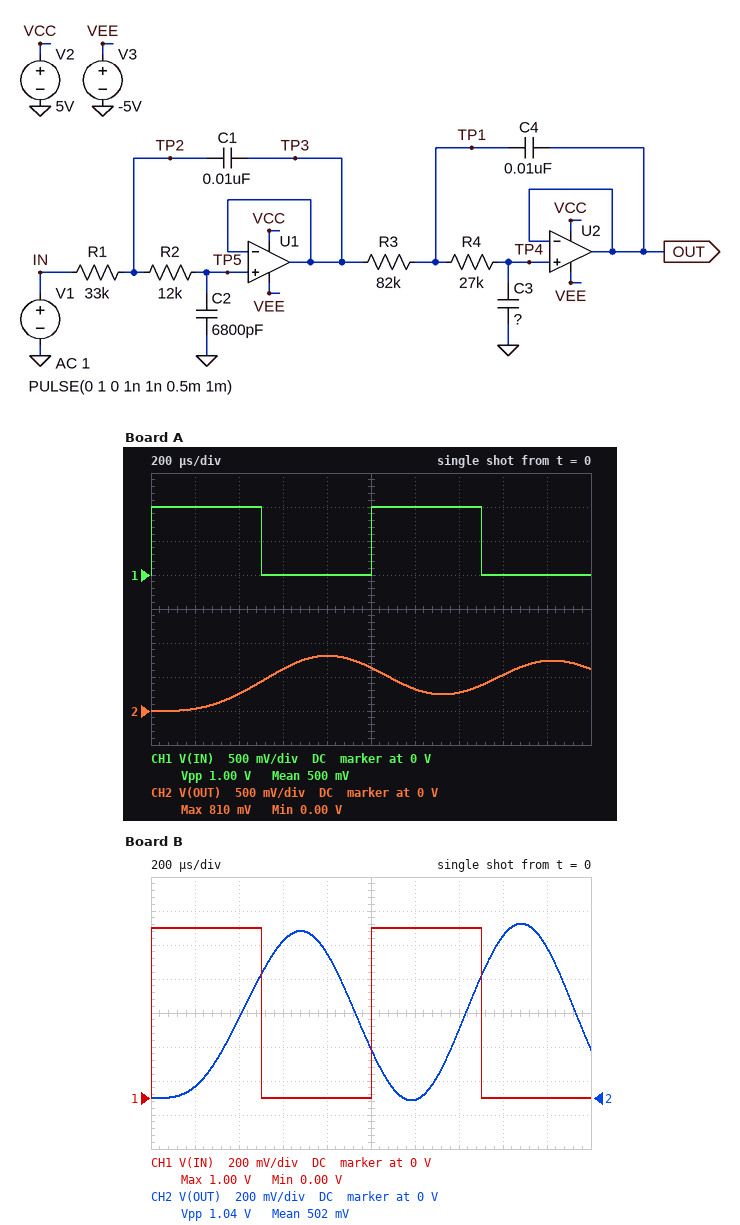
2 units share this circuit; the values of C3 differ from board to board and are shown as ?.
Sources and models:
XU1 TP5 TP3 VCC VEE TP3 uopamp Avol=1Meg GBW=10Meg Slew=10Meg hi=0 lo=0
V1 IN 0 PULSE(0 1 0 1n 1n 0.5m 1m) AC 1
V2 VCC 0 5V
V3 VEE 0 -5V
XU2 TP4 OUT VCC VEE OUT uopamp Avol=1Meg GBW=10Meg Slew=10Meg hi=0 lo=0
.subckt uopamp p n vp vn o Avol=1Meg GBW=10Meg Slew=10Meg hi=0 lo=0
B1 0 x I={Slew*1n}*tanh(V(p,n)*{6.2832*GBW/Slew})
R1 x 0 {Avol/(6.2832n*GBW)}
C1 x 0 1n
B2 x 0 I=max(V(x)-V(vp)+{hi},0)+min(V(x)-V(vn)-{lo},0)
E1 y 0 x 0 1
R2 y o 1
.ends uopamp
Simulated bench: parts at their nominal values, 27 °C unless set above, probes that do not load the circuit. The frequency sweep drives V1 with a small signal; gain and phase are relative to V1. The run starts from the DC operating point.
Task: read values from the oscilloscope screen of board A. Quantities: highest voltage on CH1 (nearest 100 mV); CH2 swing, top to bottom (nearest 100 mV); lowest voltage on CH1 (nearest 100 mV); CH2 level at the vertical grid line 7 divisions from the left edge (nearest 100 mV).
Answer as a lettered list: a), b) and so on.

a) 1.0 V
b) 800 mV
c) 0 V
d) 300 mV
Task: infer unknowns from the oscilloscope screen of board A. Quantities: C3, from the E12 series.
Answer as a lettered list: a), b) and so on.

a) 1.8 nF
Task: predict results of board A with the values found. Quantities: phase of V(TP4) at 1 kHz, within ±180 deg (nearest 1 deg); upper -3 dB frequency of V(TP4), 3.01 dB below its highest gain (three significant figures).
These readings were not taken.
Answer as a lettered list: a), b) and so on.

a) 153 deg
b) 757 Hz
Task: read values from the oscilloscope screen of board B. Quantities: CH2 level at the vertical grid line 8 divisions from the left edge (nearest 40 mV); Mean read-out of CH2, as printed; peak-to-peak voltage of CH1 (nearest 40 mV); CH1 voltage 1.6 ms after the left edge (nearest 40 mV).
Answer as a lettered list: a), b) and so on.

a) 960 mV
b) 502 mV
c) 1.00 V
d) 0 V
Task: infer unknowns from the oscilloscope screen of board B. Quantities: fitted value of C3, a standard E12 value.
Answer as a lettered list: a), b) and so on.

a) 820 pF
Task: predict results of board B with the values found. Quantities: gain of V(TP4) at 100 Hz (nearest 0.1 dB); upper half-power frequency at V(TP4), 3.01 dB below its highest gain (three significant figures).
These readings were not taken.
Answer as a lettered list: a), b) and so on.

a) 0 dB
b) 1.13 kHz
